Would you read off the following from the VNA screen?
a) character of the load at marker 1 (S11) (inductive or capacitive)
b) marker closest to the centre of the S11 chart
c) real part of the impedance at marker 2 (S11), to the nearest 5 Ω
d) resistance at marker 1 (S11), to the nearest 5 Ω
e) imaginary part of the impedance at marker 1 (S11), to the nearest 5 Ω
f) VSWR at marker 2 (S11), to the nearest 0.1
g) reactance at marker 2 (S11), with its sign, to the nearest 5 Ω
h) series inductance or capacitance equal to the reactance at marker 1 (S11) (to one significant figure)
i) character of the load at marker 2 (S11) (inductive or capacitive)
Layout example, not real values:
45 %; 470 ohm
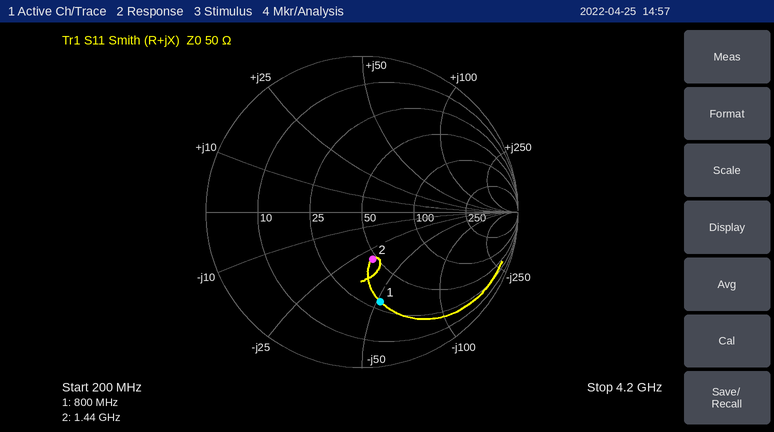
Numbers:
capacitive; marker 2; 45 Ω; 30 Ω; -50 Ω; 1.9; -30 Ω; 4 pF; capacitive
